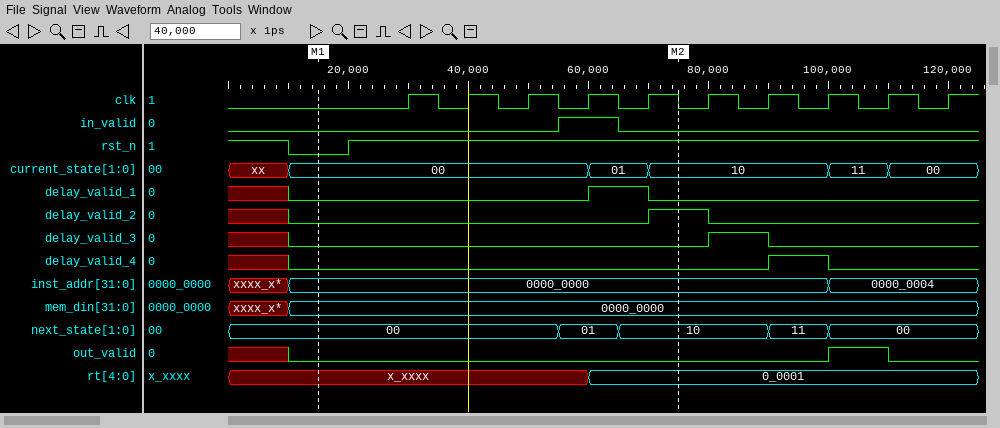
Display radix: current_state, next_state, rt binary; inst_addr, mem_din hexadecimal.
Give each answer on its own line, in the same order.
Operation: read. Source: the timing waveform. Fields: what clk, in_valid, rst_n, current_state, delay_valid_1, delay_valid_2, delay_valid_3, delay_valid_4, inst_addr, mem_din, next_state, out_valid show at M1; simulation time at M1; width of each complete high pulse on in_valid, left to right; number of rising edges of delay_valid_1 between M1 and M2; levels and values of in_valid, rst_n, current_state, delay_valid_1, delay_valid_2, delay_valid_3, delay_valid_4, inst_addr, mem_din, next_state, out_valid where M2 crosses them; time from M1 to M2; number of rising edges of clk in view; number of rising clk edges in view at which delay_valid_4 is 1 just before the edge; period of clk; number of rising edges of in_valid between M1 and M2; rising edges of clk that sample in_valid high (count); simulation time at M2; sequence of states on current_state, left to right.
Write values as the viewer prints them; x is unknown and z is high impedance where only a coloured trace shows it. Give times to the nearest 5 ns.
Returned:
clk=0, in_valid=0, rst_n=0, current_state=00, delay_valid_1=0, delay_valid_2=0, delay_valid_3=0, delay_valid_4=0, inst_addr=0000_0000, mem_din=0000_0000, next_state=00, out_valid=0
15 ns
10 ns
1
in_valid=0, rst_n=1, current_state=10, delay_valid_1=0, delay_valid_2=1, delay_valid_3=0, delay_valid_4=0, inst_addr=0000_0000, mem_din=0000_0000, next_state=10, out_valid=0
60 ns
10
1
10 ns
1
1
75 ns
xx, 00, 01, 10, 11, 00
